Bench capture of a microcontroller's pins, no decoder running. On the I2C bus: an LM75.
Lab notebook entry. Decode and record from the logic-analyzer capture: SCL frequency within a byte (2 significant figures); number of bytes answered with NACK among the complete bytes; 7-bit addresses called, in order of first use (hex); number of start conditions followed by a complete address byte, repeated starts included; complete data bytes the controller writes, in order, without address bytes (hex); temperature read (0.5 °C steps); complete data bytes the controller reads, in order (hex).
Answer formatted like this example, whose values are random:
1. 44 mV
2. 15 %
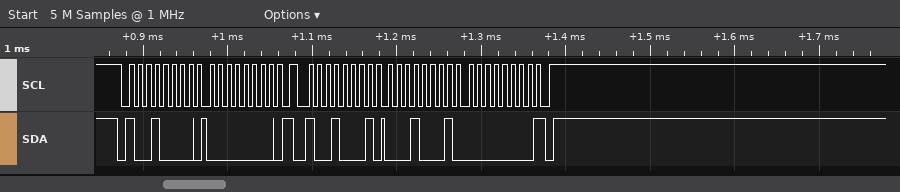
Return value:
1. 100 kHz
2. 1
3. 0x48
4. 2
5. 00
6. 17.0 °C
7. 11 00
